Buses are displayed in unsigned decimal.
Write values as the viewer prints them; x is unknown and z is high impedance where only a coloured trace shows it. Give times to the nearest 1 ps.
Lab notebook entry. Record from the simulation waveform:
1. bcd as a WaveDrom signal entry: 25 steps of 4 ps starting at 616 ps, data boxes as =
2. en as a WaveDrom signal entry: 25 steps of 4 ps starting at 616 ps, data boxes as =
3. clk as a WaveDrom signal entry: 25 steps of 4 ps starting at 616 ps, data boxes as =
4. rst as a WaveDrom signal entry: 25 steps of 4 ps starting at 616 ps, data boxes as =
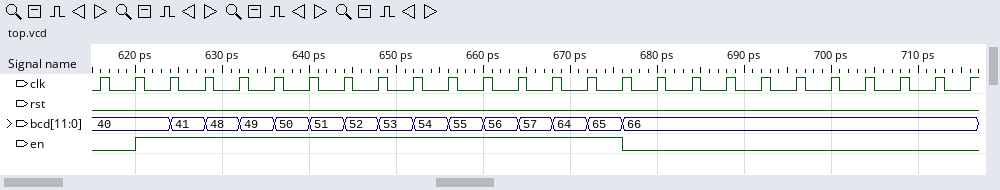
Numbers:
{name: 'bcd', wave: '=.==============.........', data: '40 41 48 49 50 51 52 53 54 55 56 57 64 65 66'}
{name: 'en', wave: '01.............0.........'}
{name: 'clk', wave: 'p........................'}
{name: 'rst', wave: '0........................'}
